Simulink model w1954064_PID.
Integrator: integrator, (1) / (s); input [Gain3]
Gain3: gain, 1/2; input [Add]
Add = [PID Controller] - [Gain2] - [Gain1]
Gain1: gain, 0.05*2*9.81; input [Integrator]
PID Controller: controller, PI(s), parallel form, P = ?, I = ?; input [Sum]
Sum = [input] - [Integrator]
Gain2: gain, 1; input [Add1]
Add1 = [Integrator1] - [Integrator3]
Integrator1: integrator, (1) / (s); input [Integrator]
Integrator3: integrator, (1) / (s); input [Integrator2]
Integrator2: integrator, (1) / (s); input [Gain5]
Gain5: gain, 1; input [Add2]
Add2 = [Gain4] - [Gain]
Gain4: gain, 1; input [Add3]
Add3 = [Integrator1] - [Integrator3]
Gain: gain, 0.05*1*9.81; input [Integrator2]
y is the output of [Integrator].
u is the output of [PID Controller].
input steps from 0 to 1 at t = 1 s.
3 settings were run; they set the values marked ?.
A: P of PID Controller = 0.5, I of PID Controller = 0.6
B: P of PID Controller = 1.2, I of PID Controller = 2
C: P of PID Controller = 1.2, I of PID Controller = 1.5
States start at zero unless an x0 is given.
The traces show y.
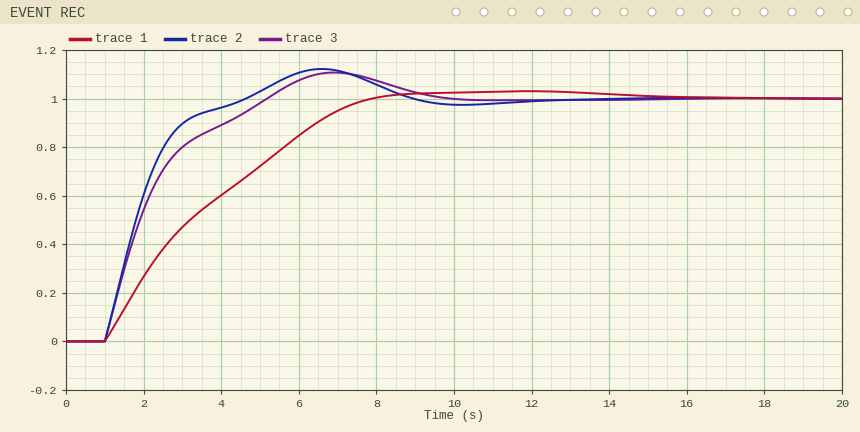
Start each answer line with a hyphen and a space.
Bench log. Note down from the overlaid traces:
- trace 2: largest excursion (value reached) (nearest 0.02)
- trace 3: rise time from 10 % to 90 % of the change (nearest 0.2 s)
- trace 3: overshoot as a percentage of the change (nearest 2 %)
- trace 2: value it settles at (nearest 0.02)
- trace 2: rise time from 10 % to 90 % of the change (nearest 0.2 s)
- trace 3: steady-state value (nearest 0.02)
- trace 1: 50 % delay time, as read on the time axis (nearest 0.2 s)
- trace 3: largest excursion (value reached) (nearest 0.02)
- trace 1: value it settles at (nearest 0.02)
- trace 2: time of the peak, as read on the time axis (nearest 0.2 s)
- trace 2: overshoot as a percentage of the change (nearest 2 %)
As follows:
- 1.12
- 3.0 s
- 10 %
- 1.00
- 1.8 s
- 1.00
- 3.2 s
- 1.10
- 1.00
- 6.6 s
- 12 %
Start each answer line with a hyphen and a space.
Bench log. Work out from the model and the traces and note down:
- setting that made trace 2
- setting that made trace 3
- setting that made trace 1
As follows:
- B
- C
- A
